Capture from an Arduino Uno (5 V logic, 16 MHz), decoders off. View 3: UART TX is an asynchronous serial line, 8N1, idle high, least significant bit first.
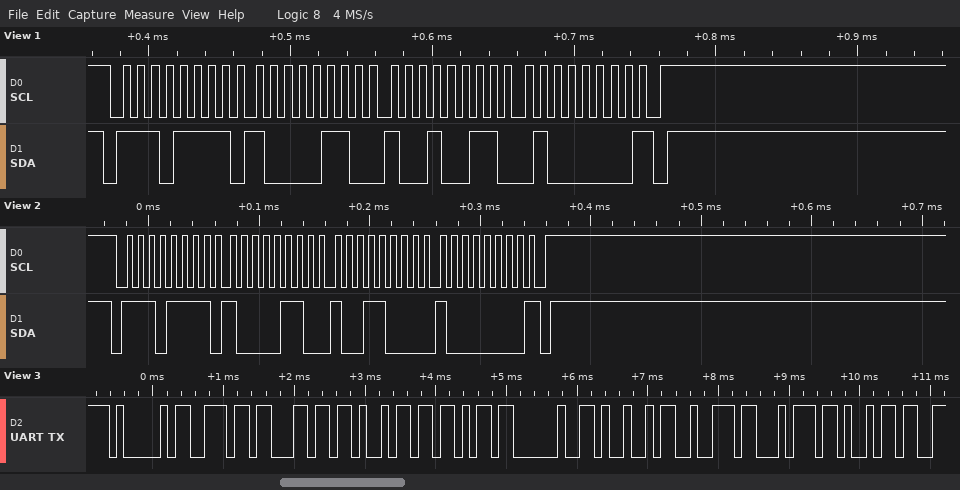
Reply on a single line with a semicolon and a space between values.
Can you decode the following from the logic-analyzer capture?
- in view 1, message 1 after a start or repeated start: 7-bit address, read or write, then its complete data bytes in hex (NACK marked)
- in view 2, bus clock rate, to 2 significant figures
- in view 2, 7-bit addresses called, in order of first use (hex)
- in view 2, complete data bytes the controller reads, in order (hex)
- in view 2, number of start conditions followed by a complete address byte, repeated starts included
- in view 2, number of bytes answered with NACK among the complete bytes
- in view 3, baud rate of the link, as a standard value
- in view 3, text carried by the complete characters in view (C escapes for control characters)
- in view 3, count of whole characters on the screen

0x77 read: 86 93 40 NACK; 100 kHz; 0x77; 86 98 80; 1; 1; 9600 baud; "Anlik Irti"; 10
